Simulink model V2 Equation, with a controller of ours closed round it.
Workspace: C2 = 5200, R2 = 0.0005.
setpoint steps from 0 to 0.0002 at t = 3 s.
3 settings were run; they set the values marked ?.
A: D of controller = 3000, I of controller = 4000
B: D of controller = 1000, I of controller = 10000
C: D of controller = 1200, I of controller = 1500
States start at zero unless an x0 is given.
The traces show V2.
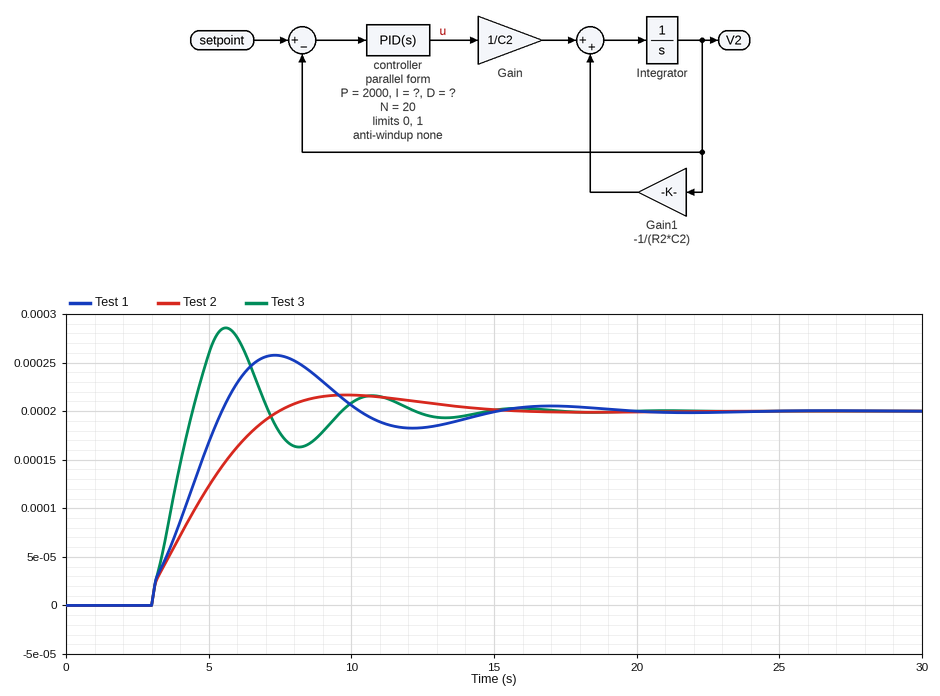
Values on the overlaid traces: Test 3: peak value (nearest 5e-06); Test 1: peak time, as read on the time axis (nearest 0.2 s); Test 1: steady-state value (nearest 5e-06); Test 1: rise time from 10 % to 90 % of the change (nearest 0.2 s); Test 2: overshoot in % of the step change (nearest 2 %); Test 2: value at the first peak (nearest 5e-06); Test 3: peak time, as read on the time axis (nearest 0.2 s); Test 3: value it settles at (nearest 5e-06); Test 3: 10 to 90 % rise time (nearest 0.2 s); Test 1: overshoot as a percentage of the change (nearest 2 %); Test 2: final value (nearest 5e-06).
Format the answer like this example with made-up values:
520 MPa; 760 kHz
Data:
0.000285; 7.4 s; 0.000200; 2.0 s; 8 %; 0.000215; 5.6 s; 0.000200; 1.2 s; 28 %; 0.000200
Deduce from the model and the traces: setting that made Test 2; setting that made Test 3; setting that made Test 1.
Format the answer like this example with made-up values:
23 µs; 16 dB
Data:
C; B; A
